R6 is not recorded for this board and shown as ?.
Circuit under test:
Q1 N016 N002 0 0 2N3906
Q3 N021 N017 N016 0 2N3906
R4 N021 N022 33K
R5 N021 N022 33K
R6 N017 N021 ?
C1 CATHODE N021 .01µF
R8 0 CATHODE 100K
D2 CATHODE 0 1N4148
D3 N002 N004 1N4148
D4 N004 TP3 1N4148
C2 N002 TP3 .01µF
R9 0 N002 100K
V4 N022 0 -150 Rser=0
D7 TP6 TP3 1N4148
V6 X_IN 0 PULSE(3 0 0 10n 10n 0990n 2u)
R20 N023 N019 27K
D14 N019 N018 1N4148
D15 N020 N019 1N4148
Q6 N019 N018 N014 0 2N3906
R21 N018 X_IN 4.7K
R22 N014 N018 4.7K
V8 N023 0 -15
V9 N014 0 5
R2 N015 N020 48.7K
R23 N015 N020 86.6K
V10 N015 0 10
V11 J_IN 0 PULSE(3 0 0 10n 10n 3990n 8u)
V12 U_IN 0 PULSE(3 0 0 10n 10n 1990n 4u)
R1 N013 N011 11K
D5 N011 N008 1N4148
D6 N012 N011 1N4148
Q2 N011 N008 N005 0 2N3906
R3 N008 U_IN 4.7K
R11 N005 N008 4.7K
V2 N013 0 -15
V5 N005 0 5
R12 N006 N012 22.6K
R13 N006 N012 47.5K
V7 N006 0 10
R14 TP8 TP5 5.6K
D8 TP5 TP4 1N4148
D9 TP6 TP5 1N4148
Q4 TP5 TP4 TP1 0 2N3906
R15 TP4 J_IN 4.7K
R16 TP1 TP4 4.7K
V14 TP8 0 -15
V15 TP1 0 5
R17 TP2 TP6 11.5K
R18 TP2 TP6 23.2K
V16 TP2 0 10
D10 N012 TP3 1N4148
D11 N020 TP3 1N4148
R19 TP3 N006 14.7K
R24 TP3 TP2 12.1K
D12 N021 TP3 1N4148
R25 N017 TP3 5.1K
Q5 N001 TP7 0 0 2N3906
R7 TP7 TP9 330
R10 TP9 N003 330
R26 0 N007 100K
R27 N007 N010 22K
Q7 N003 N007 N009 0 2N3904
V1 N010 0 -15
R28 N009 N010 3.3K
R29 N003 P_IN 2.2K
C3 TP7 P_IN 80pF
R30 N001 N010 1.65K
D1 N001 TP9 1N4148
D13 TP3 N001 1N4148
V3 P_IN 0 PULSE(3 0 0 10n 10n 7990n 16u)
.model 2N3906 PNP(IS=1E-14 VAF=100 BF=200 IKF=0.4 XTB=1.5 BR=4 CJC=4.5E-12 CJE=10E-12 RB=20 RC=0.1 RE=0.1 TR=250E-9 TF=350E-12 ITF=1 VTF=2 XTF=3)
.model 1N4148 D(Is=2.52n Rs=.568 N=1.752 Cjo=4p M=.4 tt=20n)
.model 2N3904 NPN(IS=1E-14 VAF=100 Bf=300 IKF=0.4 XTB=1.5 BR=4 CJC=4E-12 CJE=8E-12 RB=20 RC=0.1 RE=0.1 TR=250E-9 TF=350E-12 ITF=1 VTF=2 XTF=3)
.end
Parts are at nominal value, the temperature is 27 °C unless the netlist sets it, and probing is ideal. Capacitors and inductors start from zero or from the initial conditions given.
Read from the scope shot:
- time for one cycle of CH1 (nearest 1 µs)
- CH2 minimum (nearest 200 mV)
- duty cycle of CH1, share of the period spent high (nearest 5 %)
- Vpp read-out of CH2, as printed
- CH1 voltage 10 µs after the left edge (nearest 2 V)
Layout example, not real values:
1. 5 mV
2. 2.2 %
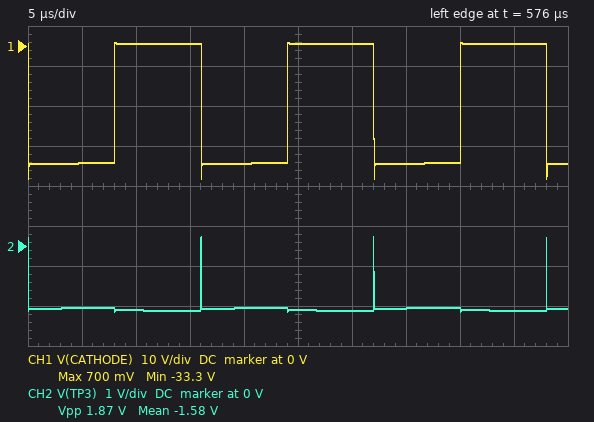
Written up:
1. 16 µs
2. -1.6 V
3. 50 %
4. 1.87 V
5. 0 V
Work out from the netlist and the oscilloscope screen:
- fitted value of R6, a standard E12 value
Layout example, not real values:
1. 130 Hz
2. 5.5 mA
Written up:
1. 1.8 kΩ
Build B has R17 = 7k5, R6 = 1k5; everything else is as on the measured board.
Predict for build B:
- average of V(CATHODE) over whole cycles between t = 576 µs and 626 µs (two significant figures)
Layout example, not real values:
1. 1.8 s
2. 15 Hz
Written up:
1. -15 V
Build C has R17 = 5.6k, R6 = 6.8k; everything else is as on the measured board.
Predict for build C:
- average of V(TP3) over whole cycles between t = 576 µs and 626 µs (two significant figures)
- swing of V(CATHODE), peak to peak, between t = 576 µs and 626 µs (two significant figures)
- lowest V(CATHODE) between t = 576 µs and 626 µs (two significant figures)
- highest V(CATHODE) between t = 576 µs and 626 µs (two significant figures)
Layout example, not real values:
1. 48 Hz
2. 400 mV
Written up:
1. -1.2 V
2. 59 V
3. -58 V
4. 720 mV
